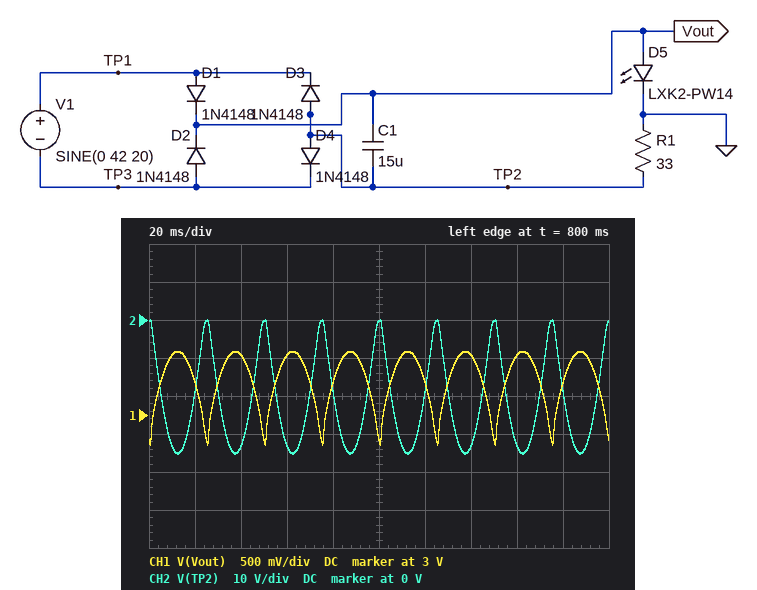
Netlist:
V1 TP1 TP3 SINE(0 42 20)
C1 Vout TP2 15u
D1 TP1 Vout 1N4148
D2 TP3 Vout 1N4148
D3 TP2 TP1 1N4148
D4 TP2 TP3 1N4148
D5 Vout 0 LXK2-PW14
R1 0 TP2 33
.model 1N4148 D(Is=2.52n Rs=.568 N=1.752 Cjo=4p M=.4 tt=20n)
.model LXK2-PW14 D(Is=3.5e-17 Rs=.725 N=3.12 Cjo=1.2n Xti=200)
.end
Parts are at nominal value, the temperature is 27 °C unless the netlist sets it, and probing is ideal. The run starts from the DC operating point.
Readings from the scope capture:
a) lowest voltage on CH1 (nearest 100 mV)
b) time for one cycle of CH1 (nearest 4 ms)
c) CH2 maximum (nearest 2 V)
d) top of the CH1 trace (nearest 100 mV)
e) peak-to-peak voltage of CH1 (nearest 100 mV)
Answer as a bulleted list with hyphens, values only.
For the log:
- 2.6 V
- 24 ms
- 0 V
- 3.8 V
- 1.2 V
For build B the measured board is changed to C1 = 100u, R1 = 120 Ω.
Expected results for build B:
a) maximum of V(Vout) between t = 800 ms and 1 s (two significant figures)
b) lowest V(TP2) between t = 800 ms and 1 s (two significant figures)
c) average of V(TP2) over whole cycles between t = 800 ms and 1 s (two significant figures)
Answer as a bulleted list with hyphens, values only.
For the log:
- 3.2 V
- -37 V
- -26 V
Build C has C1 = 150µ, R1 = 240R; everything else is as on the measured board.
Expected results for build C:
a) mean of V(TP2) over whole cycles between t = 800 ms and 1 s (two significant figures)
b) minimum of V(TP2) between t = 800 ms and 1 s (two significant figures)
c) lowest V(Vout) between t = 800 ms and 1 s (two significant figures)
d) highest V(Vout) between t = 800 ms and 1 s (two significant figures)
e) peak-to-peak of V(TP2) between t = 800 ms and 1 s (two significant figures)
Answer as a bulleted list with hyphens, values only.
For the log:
- -31 V
- -37 V
- 2.9 V
- 3.0 V
- 14 V
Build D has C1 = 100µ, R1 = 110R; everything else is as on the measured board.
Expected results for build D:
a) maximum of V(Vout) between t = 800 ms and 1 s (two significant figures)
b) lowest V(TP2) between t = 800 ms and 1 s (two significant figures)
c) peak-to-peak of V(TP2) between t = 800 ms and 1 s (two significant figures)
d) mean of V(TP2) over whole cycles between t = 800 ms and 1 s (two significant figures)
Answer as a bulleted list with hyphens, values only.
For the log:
- 3.2 V
- -37 V
- 25 V
- -25 V
